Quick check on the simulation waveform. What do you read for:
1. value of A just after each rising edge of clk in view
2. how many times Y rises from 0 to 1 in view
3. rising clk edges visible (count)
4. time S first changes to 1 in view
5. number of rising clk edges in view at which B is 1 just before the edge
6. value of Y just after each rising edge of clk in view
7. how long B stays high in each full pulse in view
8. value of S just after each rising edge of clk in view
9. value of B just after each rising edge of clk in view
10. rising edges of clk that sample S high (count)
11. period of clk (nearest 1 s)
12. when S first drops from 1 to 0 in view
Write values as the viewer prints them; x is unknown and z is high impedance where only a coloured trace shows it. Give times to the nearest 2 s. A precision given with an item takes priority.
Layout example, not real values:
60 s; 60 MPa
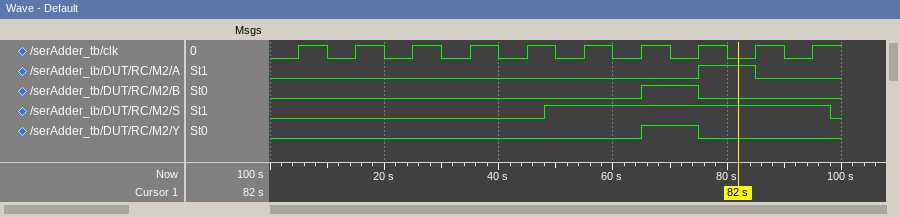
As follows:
0 0 0 0 0 0 0 1 0 0; 1; 10; 48 s; 1; 0 0 0 0 0 0 1 0 0 0; 10 s; 0 0 0 0 0 1 1 1 1 1; 0 0 0 0 0 0 1 0 0 0; 5; 10 s; 98 s
